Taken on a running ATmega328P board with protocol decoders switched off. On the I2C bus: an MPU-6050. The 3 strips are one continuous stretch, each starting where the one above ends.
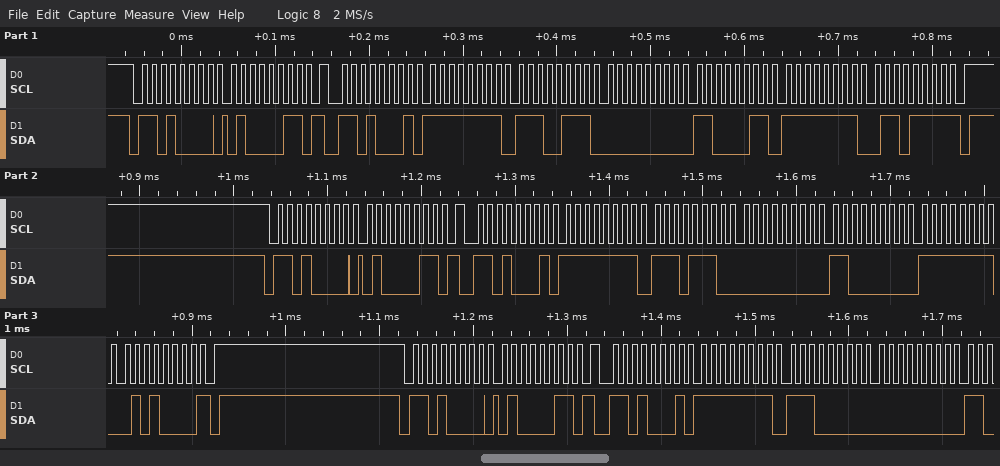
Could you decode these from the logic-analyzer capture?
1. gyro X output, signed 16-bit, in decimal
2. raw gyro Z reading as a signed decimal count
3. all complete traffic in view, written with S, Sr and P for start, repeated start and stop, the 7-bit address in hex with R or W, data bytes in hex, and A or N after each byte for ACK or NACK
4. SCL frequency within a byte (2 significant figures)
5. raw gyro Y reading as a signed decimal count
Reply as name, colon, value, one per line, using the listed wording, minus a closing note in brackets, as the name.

gyro X output, signed 16-bit, in decimal: -25
raw gyro Z reading as a signed decimal count: -145
all complete traffic in view, written with S, Sr and P for start, repeated start and stop, the 7-bit address in hex with R or W, data bytes in hex, and A or N after each byte for ACK or NACK: S 68W A 43 A Sr 68R A FF A E7 A 00 A C3 A FF A 6F N P S 68W A 43 A Sr 68R A FF A EE A 00 A C0 A FF A 50 N P S 68W A 43 A Sr 68R A FF A E0 A 00 A
SCL frequency within a byte: 100 kHz
raw gyro Y reading as a signed decimal count: 195
